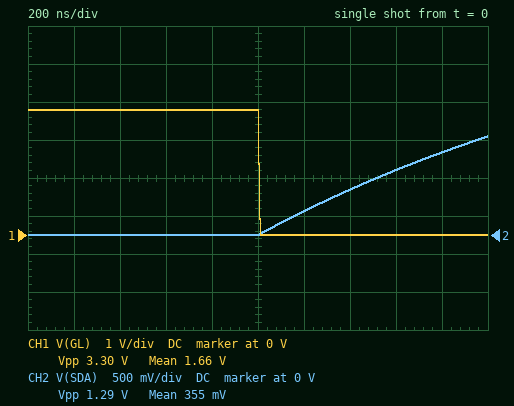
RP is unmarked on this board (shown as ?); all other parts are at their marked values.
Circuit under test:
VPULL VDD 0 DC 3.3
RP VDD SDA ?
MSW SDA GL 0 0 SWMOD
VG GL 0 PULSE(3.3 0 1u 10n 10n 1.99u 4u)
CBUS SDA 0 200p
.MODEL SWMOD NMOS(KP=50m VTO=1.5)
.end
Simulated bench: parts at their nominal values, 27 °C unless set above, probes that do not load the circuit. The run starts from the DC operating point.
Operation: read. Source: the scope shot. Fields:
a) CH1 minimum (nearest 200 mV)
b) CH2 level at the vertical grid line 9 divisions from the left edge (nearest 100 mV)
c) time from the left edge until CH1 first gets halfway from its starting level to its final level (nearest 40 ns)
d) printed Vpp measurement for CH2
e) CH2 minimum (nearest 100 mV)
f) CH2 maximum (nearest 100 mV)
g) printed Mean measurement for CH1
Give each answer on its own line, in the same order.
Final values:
0 V
1.1 V
1.00 µs
1.29 V
0 V
1.3 V
1.66 V
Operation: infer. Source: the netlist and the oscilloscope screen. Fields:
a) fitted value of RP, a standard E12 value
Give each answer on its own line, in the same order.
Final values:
10 kΩ
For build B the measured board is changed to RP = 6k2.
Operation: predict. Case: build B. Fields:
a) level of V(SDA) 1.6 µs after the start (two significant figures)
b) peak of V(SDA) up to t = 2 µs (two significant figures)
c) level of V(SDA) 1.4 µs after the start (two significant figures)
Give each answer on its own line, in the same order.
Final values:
1.3 V
1.8 V
910 mV
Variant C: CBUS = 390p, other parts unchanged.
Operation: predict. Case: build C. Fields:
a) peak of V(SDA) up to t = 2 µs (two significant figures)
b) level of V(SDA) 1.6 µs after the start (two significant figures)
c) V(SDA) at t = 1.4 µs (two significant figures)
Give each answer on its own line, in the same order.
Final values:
750 mV
470 mV
320 mV
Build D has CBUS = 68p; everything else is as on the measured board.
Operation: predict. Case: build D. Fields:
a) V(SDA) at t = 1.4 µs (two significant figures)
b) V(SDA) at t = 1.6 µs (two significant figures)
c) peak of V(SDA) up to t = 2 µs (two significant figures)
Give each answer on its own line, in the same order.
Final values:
1.5 V
1.9 V
2.5 V
